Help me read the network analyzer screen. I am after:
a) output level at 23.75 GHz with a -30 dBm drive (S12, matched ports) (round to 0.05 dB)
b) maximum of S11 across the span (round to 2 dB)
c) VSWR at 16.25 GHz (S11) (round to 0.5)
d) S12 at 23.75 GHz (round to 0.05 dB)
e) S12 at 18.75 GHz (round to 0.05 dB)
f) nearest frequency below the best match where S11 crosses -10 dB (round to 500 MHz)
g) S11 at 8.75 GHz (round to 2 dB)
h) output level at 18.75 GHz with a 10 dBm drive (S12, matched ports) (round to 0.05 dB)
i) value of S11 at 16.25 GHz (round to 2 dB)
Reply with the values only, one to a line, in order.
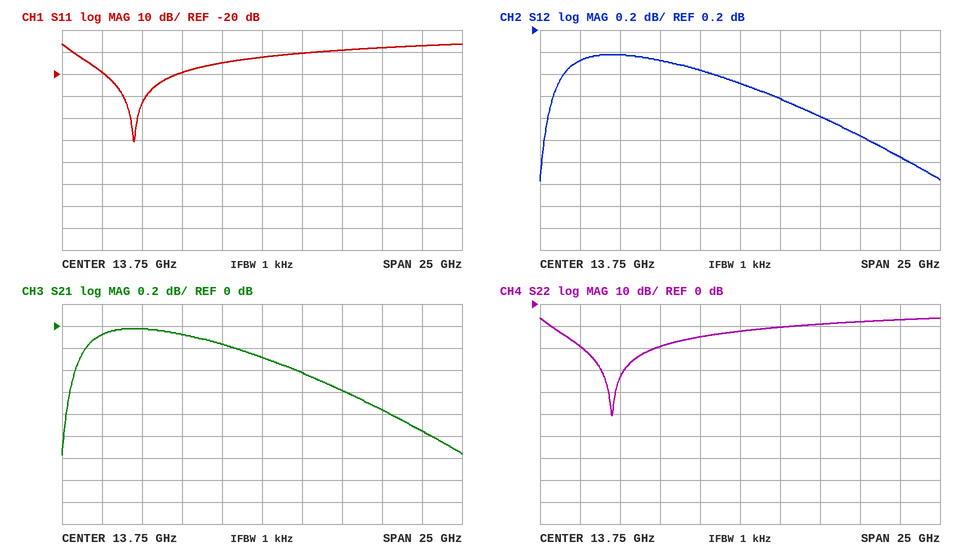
-30.95 dBm
-6 dB
2.0
-0.95 dB
-0.60 dB
2.0 GHz
-20 dB
9.40 dBm
-10 dB
